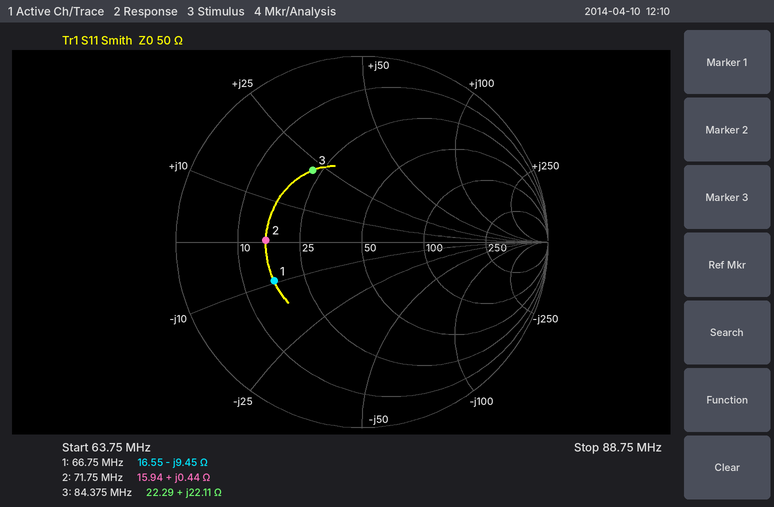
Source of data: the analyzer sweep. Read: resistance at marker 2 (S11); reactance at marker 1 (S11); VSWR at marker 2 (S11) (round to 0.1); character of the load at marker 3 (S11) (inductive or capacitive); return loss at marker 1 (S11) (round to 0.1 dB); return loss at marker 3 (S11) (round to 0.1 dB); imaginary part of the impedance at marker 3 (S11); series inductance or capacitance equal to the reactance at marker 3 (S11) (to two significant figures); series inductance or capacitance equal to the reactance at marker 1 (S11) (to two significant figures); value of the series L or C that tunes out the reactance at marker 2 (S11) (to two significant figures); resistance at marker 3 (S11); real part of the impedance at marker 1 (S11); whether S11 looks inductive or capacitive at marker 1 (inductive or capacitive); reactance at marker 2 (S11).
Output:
15.94 Ω
-9.45 Ω
3.1
inductive
5.7 dB
6.6 dB
+22.11 Ω
42 nH
250 pF
5.0 nF
22.29 Ω
16.55 Ω
capacitive
+0.44 Ω
